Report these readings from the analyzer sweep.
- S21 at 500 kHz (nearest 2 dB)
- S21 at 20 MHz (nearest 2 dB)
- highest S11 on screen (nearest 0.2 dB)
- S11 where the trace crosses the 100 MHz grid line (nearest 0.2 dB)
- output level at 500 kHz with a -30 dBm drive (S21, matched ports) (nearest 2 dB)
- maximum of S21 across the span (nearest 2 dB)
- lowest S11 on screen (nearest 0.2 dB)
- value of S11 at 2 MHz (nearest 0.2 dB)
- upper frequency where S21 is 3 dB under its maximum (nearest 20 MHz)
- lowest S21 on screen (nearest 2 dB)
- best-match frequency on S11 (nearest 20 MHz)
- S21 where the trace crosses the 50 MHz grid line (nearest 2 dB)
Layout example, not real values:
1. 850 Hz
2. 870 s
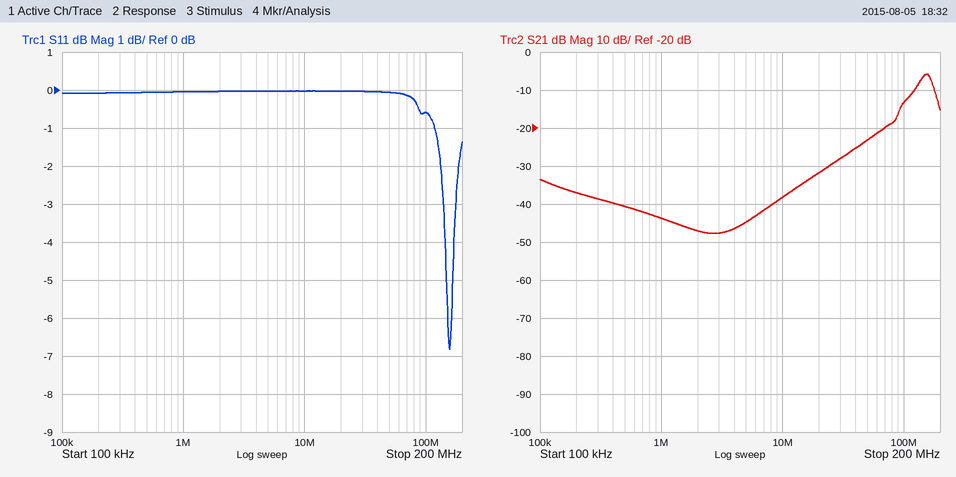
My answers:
1. -40 dB
2. -32 dB
3. 0.0 dB
4. -0.6 dB
5. -70 dBm
6. -6 dB
7. -6.8 dB
8. 0.0 dB
9. 180 MHz
10. -48 dB
11. 160 MHz
12. -24 dB
